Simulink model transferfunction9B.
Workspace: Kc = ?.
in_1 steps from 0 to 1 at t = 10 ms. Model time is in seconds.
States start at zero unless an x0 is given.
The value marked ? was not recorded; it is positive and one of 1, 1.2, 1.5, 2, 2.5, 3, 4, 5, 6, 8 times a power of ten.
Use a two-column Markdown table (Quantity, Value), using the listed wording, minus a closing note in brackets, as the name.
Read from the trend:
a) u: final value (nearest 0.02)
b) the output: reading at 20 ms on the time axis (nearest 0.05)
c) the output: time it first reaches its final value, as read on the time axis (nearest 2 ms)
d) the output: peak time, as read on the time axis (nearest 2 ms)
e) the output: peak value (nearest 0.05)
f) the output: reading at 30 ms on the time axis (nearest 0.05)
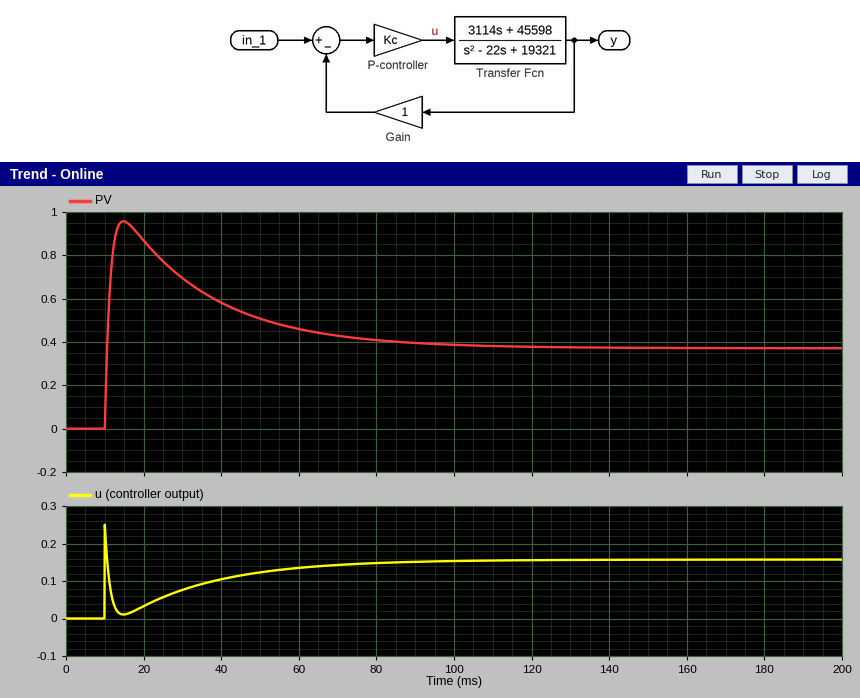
| Quantity | Value |
|---|---|
| u: final value | 0.16 |
| the output: reading at 20 ms on the time axis | 0.85 |
| the output: time it first reaches its final value, as read on the time axis | 10 ms |
| the output: peak time, as read on the time axis | 14 ms |
| the output: peak value | 0.95 |
| the output: reading at 30 ms on the time axis | 0.70 |
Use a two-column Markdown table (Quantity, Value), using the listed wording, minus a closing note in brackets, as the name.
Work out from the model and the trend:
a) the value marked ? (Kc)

| Quantity | Value |
|---|---|
| the value marked ? | 0.25 |
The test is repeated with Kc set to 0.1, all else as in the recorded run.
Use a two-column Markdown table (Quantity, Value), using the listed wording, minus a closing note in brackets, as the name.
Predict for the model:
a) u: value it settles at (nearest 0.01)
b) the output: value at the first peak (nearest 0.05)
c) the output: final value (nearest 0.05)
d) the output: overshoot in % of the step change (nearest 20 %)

| Quantity | Value |
|---|---|
| u: value it settles at | 0.08 |
| the output: value at the first peak | 0.85 |
| the output: final value | 0.20 |
| the output: overshoot in % of the step change | 340 % |
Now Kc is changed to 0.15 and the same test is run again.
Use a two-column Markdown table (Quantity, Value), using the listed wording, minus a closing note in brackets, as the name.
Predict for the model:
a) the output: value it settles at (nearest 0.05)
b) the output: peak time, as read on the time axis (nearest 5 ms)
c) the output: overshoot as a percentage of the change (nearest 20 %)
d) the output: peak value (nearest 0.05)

| Quantity | Value |
|---|---|
| the output: value it settles at | 0.25 |
| the output: peak time, as read on the time axis | 15 ms |
| the output: overshoot as a percentage of the change | 240 % |
| the output: peak value | 0.90 |
